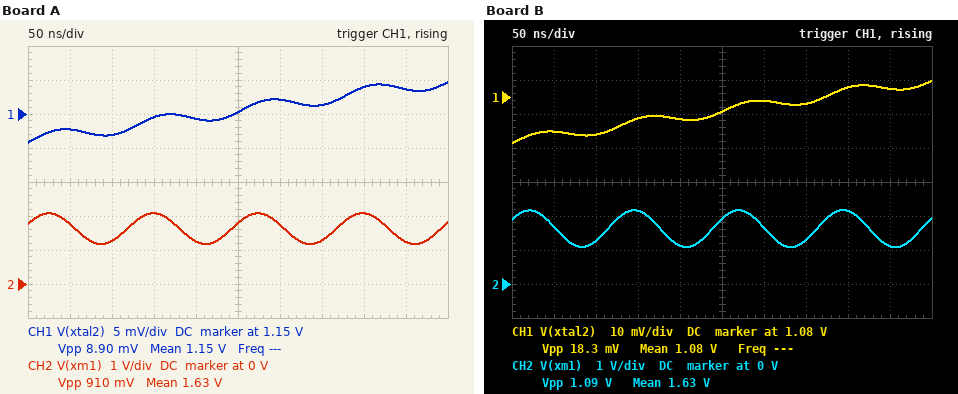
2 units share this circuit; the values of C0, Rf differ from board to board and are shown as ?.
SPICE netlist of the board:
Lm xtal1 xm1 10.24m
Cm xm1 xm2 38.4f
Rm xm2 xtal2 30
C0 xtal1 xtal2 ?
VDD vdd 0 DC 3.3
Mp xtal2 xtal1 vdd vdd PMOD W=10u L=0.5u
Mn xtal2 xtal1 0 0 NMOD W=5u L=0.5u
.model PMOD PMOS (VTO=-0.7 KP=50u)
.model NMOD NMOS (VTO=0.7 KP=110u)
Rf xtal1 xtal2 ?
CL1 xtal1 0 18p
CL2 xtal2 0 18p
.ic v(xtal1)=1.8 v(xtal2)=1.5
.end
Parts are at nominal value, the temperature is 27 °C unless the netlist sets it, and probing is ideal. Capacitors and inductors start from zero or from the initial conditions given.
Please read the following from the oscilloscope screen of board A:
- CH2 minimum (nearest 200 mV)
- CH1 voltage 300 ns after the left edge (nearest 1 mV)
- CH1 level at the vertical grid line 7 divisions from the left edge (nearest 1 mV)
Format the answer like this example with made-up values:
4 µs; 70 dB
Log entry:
1.2 V; 1.152 V; 1.151 V
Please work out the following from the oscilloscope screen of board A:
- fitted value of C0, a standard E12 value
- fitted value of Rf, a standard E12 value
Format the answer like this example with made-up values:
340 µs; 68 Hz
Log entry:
10 pF; 2.7 MΩ
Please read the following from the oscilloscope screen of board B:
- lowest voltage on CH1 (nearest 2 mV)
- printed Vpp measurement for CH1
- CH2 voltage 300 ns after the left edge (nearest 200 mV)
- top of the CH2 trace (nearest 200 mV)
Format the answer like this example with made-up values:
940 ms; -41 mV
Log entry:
1.066 V; 18.3 mV; 1.6 V; 2.2 V
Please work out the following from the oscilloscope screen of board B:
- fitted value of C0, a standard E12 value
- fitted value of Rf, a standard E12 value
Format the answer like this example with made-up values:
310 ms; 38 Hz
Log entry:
5.6 pF; 2.7 MΩ
